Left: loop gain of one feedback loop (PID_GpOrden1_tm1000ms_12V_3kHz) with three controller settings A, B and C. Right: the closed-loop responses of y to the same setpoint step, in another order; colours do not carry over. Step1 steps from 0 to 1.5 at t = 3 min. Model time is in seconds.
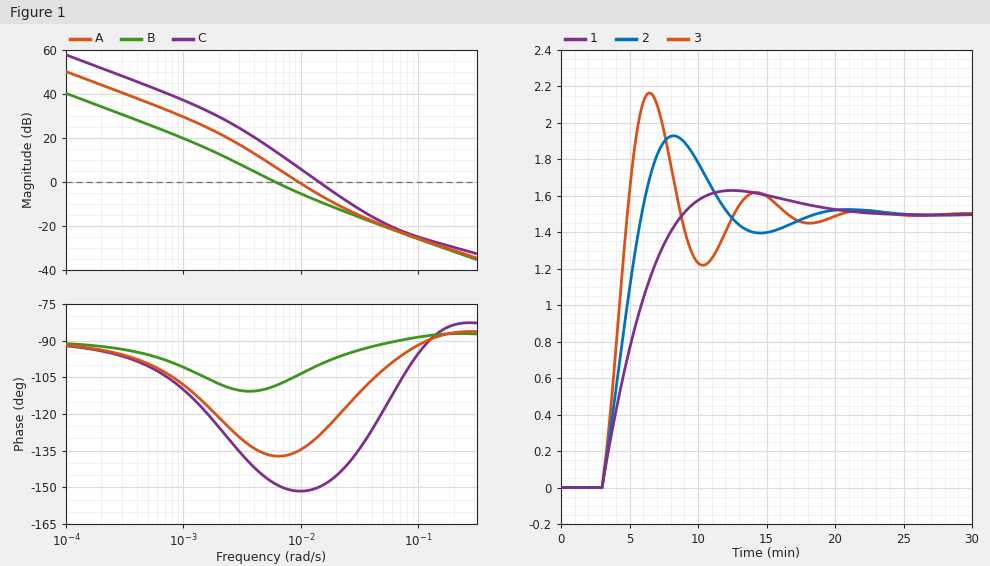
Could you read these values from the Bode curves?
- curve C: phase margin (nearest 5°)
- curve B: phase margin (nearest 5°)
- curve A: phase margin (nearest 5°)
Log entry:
30°
70°
45°
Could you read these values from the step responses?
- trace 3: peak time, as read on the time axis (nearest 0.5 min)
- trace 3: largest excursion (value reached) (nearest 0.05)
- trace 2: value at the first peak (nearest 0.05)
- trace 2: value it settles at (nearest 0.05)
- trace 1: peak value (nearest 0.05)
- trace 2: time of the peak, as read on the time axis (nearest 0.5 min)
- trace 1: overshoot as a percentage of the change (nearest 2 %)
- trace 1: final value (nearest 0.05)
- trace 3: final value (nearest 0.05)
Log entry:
6.5 min
2.15
1.95
1.50
1.65
8.0 min
8 %
1.50
1.50
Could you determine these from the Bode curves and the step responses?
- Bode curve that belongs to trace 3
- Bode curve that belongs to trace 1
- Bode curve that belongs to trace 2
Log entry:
C
B
A
